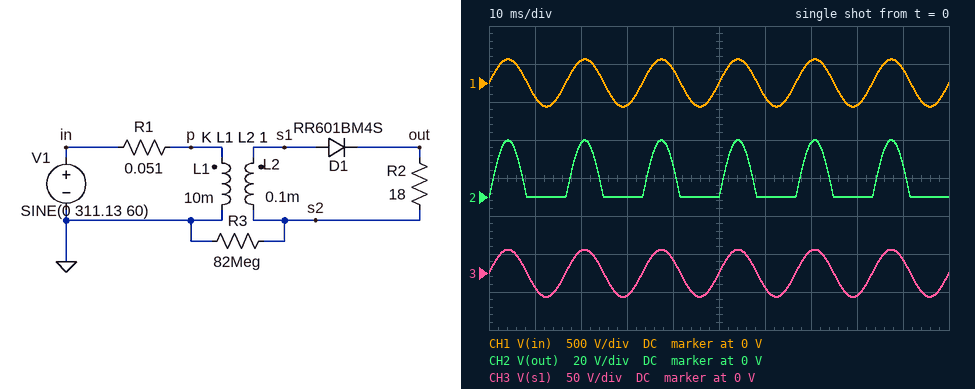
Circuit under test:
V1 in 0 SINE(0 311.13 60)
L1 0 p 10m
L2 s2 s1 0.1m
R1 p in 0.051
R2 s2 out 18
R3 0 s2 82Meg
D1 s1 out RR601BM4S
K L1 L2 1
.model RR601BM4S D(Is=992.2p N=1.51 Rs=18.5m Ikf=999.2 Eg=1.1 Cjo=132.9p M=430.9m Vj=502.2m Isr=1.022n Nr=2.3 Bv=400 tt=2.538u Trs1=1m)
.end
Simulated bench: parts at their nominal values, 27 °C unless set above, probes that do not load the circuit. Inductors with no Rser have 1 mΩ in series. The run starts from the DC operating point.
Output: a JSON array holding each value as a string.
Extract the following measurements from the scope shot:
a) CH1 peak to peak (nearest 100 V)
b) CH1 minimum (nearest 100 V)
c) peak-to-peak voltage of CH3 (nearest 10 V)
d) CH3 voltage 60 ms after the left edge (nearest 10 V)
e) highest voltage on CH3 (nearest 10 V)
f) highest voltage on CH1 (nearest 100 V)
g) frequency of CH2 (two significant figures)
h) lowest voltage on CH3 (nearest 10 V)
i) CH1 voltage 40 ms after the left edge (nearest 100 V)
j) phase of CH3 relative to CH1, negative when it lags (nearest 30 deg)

["600 V", "-300 V", "60 V", "-20 V", "30 V", "300 V", "60 Hz", "-30 V", "200 V", "0 deg"]
